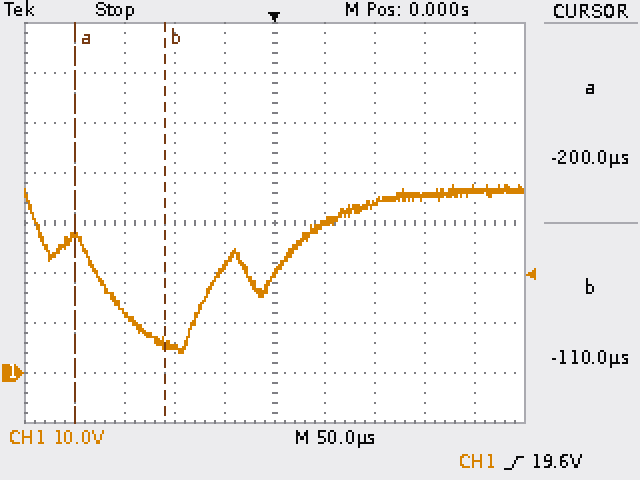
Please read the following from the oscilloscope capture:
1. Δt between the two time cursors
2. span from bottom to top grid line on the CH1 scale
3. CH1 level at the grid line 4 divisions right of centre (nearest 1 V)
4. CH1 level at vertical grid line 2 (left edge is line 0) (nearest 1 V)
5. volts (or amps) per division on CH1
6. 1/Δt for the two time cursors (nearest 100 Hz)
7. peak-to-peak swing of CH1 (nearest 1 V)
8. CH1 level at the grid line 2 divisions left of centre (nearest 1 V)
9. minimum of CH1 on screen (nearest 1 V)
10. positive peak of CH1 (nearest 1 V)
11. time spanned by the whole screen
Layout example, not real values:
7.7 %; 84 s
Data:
90 µs; 80 V; 37 V; 12 V; 10 V; 11.1 kHz; 34 V; 5 V; 4 V; 38 V; 500 µs
